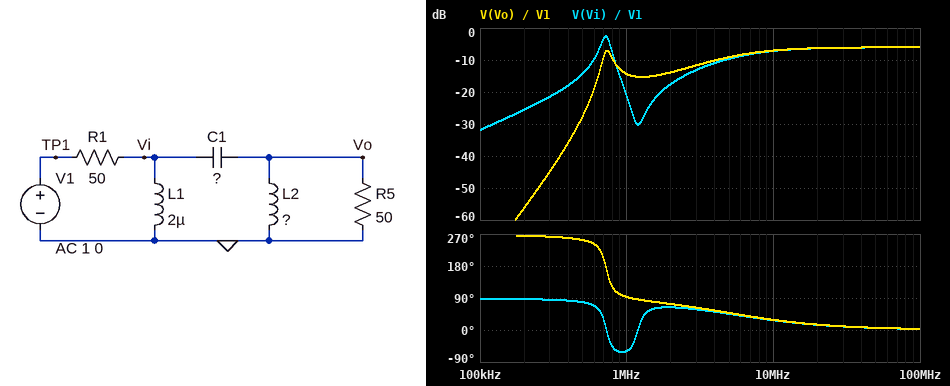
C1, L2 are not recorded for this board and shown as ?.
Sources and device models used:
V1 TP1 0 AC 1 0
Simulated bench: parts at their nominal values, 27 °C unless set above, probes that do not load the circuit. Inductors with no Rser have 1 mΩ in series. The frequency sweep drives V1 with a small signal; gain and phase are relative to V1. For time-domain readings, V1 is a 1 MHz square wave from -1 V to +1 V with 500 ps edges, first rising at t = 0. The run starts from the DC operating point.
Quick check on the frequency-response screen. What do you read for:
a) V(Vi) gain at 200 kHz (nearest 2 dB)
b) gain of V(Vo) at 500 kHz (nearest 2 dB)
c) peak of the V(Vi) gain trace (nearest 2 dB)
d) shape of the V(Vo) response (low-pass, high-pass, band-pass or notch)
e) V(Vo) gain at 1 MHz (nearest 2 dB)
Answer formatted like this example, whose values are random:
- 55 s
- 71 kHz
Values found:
- -26 dB
- -28 dB
- -2 dB
- high-pass
- -14 dB
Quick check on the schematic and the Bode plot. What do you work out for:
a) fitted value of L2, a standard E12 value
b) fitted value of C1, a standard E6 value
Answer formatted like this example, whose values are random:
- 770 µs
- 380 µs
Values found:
- 1.2 µH
- 15 nF
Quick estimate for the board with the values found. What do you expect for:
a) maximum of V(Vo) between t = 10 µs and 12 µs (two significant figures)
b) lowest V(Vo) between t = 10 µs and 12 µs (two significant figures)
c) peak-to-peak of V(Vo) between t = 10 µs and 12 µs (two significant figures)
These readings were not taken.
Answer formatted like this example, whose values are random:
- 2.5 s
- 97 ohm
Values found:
- 1.1 V
- -1.1 V
- 2.3 V
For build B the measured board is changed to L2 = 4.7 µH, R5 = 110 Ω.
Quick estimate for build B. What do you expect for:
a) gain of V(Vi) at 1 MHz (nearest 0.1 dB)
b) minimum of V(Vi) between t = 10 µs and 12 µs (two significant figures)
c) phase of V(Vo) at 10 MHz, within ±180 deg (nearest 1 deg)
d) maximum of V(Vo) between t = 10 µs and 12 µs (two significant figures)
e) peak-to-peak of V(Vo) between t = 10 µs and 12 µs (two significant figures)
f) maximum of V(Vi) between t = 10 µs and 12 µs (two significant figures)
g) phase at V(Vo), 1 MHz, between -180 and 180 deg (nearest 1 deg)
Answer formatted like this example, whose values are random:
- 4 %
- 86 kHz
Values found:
- -16.6 dB
- -1.3 V
- 22 deg
- 1.5 V
- 2.9 V
- 1.3 V
- 81 deg
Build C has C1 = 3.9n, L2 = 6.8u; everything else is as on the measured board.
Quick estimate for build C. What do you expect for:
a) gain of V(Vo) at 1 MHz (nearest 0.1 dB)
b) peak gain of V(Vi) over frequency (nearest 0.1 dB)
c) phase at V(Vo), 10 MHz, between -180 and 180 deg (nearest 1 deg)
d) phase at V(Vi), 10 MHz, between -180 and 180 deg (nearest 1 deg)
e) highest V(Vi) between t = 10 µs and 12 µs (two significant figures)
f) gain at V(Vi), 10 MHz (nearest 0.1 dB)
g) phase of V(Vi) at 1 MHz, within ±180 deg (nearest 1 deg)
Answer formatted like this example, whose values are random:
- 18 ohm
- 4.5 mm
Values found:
- -9.8 dB
- -6.0 dB
- 17 deg
- 12 deg
- 990 mV
- -6.3 dB
- 49 deg
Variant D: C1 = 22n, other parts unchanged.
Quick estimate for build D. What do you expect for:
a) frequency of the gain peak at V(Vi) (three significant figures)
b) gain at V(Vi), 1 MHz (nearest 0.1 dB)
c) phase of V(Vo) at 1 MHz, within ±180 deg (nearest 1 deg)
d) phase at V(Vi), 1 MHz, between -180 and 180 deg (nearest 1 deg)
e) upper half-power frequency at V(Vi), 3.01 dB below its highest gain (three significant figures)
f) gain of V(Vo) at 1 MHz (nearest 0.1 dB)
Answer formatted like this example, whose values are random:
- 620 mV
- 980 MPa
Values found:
- 597 kHz
- -33.3 dB
- 86 deg
- 12 deg
- 634 kHz
- -16.8 dB
